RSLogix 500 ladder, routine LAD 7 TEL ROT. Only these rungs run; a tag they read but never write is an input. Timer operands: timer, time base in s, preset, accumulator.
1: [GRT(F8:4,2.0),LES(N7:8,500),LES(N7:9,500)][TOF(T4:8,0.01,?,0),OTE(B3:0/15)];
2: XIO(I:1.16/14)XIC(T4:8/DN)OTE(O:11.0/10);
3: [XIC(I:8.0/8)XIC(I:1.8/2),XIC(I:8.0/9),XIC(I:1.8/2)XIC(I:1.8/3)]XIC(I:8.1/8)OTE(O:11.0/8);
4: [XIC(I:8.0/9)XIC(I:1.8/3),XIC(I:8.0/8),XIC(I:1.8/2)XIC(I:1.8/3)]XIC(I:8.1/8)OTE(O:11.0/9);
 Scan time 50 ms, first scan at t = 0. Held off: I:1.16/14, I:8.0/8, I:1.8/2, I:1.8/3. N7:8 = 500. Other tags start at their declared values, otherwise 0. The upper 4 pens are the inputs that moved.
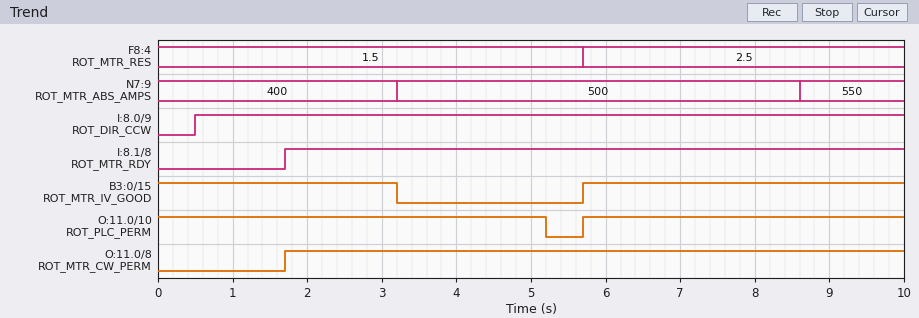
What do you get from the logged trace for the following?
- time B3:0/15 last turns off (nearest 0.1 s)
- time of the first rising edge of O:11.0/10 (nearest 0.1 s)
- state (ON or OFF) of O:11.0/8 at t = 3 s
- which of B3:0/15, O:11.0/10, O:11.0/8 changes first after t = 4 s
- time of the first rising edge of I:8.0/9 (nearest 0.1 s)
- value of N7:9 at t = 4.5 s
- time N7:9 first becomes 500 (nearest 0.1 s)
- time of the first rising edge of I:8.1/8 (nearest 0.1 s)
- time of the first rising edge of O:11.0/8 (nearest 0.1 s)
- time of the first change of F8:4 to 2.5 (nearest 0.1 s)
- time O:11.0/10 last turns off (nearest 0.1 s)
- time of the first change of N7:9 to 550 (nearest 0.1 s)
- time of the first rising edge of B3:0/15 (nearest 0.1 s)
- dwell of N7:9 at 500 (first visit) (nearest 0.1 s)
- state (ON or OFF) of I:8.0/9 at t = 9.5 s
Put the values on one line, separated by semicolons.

3.2 s; 5.7 s; ON; O:11.0/10; 0.5 s; 500; 3.2 s; 1.7 s; 1.7 s; 5.7 s; 5.2 s; 8.6 s; 5.7 s; 5.4 s; ON
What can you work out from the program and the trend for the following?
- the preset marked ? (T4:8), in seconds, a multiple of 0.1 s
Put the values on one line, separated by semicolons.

2.0 s
